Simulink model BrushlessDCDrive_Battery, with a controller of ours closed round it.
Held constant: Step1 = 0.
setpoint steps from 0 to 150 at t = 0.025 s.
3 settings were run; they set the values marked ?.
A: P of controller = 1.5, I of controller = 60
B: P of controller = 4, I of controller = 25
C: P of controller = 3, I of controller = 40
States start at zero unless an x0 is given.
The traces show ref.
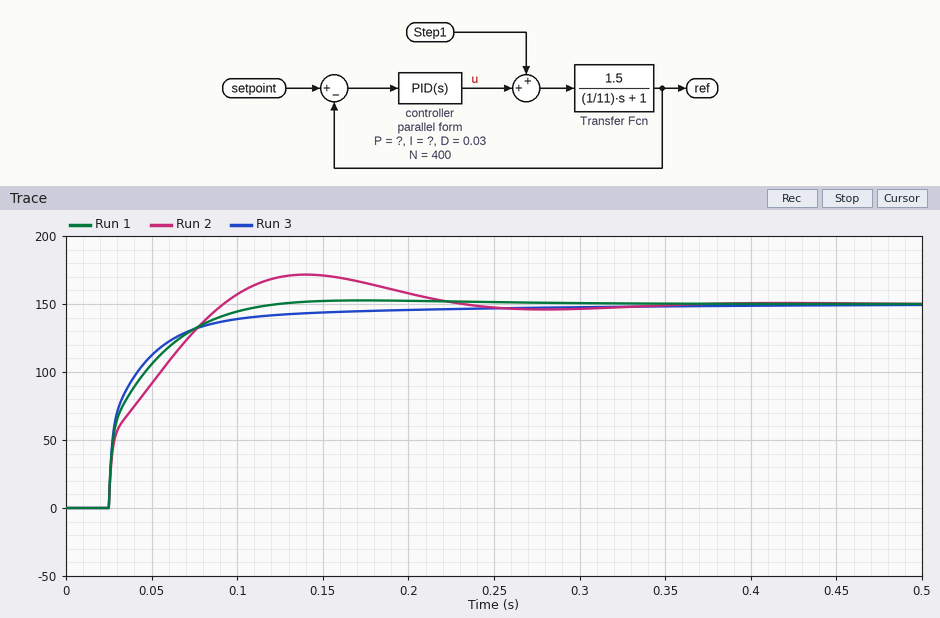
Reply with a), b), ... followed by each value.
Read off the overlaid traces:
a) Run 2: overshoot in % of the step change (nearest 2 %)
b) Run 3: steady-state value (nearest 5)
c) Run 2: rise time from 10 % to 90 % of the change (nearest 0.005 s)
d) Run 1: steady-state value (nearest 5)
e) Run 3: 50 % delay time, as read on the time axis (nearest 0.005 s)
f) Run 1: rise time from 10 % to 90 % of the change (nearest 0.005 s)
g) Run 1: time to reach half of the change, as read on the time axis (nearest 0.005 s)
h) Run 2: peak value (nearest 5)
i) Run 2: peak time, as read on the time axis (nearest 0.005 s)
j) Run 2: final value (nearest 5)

a) 14 %
b) 150
c) 0.055 s
d) 150
e) 0.030 s
f) 0.055 s
g) 0.035 s
h) 170
i) 0.140 s
j) 150
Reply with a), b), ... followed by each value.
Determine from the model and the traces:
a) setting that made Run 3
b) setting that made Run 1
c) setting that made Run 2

a) B
b) C
c) A
